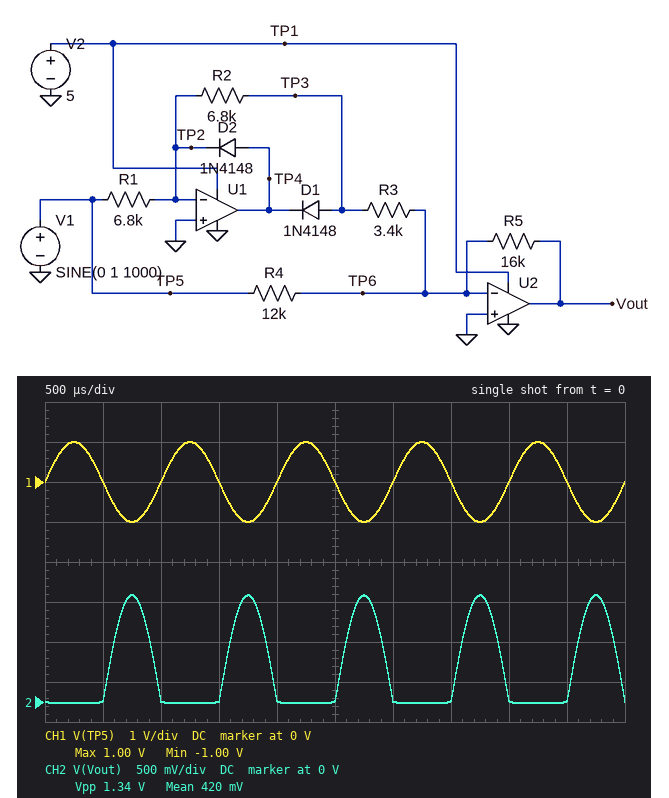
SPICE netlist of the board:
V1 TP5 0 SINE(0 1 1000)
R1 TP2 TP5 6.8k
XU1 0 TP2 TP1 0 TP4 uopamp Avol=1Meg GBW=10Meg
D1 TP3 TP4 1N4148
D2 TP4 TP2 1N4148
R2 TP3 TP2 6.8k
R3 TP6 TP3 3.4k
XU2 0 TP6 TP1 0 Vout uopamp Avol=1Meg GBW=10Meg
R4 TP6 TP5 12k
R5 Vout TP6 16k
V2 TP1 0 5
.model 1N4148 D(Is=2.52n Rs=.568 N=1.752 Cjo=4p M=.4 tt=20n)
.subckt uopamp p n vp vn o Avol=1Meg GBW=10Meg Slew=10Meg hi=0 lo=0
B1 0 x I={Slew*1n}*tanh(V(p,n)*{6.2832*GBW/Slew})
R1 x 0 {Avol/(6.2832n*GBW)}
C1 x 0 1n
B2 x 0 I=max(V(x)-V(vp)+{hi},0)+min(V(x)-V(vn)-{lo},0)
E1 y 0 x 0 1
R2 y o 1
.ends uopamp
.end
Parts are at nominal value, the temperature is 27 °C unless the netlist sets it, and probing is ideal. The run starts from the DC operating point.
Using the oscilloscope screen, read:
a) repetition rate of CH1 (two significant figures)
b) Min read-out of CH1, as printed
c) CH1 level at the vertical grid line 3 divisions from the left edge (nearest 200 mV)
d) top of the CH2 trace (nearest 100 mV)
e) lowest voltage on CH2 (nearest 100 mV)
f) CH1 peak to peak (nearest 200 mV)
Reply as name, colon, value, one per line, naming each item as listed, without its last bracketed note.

repetition rate of CH1: 1.0 kHz
Min read-out of CH1, as printed: -1.00 V
CH1 level at the vertical grid line 3 divisions from the left edge: 0 V
top of the CH2 trace: 1.3 V
lowest voltage on CH2: 0 V
CH1 peak to peak: 2.0 V
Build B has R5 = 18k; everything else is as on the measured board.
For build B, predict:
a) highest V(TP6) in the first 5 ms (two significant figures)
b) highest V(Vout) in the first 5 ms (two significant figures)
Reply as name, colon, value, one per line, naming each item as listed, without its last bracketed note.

highest V(TP6) in the first 5 ms: 490 mV
highest V(Vout) in the first 5 ms: 1.5 V
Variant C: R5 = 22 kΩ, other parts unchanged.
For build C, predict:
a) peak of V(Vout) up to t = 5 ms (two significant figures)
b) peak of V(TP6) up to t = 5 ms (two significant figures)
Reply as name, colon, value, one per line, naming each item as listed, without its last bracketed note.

peak of V(Vout) up to t = 5 ms: 1.8 V
peak of V(TP6) up to t = 5 ms: 510 mV
